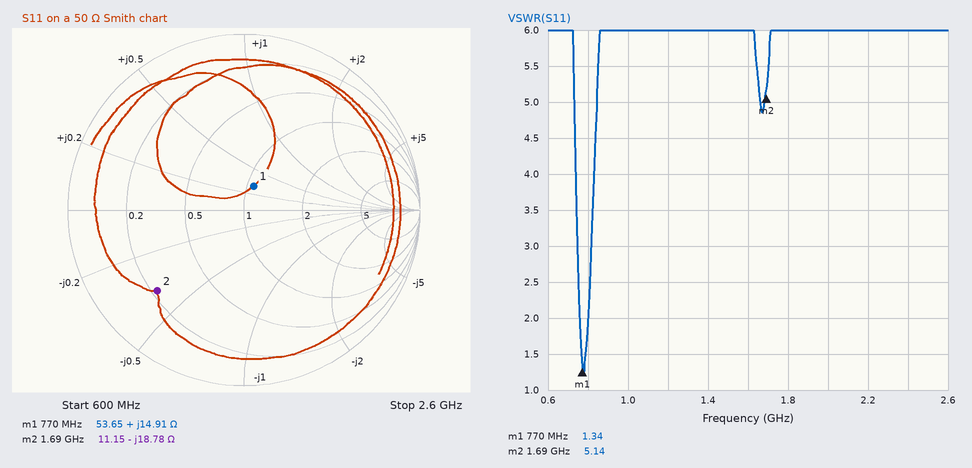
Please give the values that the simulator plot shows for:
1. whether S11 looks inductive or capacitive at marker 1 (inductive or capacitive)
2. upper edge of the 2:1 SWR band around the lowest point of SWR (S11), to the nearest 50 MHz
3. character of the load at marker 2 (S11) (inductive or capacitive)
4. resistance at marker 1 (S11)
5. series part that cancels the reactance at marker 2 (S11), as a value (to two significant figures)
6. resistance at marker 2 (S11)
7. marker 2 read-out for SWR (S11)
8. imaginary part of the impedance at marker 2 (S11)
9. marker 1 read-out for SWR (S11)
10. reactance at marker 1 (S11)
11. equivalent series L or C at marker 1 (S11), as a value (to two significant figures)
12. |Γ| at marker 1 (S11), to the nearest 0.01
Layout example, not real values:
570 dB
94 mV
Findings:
inductive
800 MHz
capacitive
53.65 Ω
1.8 nH
11.15 Ω
5.14
-18.78 Ω
1.34
+14.91 Ω
3.1 nH
0.15
